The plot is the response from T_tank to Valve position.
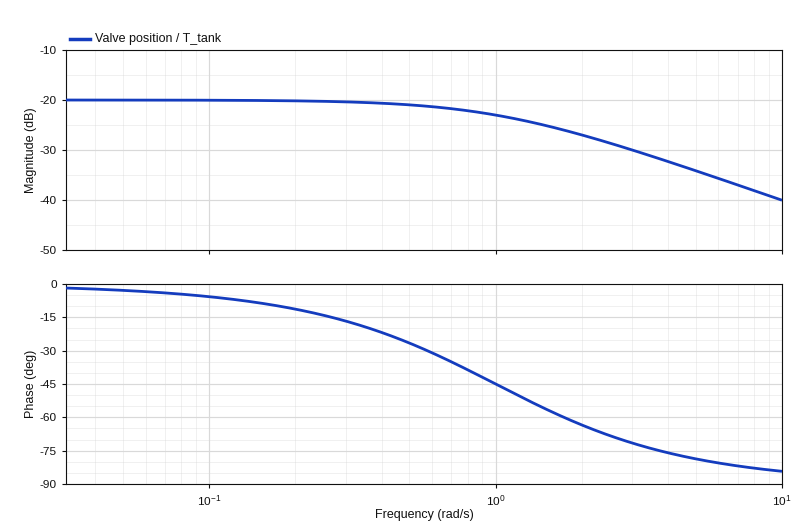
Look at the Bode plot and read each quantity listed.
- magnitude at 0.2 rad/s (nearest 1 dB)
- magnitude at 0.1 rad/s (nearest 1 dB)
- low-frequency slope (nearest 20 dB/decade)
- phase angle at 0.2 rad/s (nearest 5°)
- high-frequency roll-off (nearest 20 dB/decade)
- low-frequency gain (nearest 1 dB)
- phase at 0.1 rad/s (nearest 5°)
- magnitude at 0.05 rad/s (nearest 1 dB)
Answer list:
-20 dB
-20 dB
0 dB/decade
-10°
-20 dB/decade
-20 dB
-5°
-20 dB
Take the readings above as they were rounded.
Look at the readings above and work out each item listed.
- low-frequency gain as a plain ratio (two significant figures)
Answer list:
0.10
